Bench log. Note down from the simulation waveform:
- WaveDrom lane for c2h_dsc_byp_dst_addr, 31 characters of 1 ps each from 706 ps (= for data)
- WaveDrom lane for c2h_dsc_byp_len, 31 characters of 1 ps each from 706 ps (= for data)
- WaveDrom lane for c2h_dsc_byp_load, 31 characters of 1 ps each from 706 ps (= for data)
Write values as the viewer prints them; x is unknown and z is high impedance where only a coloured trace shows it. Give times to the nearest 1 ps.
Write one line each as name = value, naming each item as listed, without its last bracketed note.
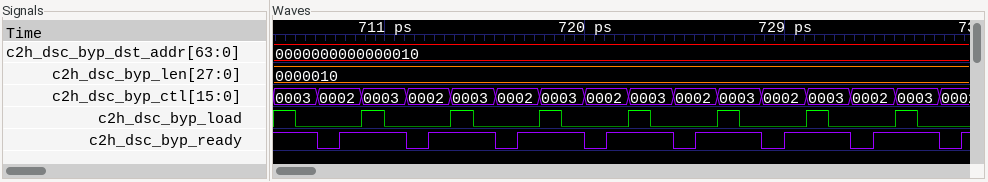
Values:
WaveDrom lane for c2h_dsc_byp_dst_addr, 31 characters of 1 ps each from 706 ps = {name: 'c2h_dsc_byp_dst_addr', wave: '=..............................', data: '0000000000000010'}
WaveDrom lane for c2h_dsc_byp_len, 31 characters of 1 ps each from 706 ps = {name: 'c2h_dsc_byp_len', wave: '=..............................', data: '0000010'}
WaveDrom lane for c2h_dsc_byp_load, 31 characters of 1 ps each from 706 ps = {name: 'c2h_dsc_byp_load', wave: '10..10..10..10..10..10..10..10.'}
